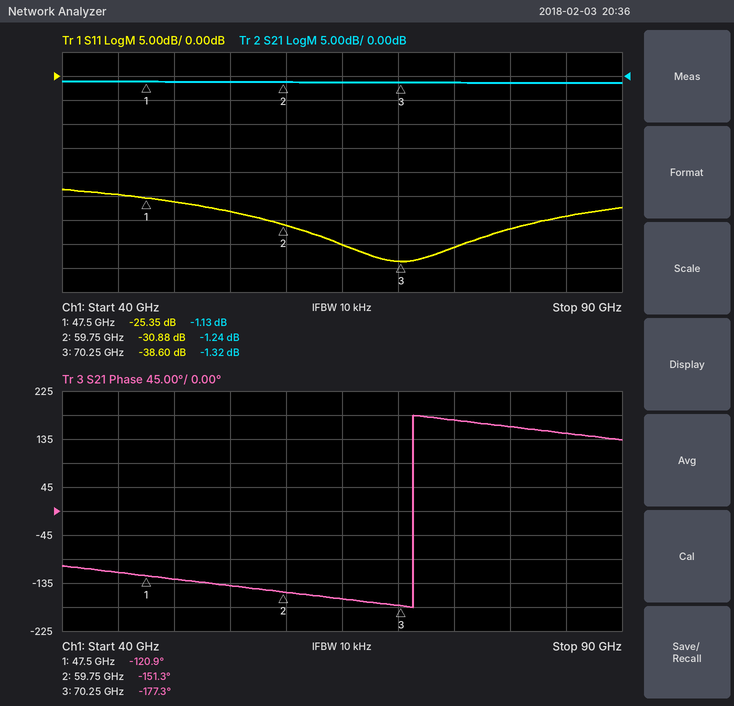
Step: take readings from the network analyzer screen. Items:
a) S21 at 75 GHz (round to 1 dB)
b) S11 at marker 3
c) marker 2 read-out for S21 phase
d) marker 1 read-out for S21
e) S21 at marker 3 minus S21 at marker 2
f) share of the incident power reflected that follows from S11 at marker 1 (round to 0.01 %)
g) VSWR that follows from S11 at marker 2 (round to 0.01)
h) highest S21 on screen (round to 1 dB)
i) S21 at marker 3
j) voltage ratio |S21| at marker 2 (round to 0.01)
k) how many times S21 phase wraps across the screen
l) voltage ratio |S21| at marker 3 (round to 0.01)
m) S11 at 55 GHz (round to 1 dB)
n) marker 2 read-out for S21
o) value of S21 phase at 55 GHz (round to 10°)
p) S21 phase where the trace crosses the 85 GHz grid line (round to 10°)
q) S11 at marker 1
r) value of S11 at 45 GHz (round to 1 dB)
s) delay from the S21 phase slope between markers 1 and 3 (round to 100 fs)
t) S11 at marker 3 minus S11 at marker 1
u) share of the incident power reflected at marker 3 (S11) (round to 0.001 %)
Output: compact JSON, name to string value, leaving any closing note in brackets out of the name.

{"S21 at 75 GHz": "-1 dB", "S11 at marker 3": "-38.60 dB", "marker 2 read-out for S21 phase": "-151.3°", "marker 1 read-out for S21": "-1.13 dB", "S21 at marker 3 minus S21 at marker 2": "-0.08 dB", "share of the incident power reflected that follows from S11 at marker 1": "0.29 %", "VSWR that follows from S11 at marker 2": "1.06", "highest S21 on screen": "-1 dB", "S21 at marker 3": "-1.32 dB", "voltage ratio |S21| at marker 2": "0.87", "how many times S21 phase wraps across the screen": "1", "voltage ratio |S21| at marker 3": "0.86", "S11 at 55 GHz": "-28 dB", "marker 2 read-out for S21": "-1.24 dB", "value of S21 phase at 55 GHz": "-140°", "S21 phase where the trace crosses the 85 GHz grid line": "150°", "S11 at marker 1": "-25.35 dB", "value of S11 at 45 GHz": "-25 dB", "delay from the S21 phase slope between markers 1 and 3": "6.9 ps", "S11 at marker 3 minus S11 at marker 1": "-13.25 dB", "share of the incident power reflected at marker 3 (S11)": "0.014 %"}
